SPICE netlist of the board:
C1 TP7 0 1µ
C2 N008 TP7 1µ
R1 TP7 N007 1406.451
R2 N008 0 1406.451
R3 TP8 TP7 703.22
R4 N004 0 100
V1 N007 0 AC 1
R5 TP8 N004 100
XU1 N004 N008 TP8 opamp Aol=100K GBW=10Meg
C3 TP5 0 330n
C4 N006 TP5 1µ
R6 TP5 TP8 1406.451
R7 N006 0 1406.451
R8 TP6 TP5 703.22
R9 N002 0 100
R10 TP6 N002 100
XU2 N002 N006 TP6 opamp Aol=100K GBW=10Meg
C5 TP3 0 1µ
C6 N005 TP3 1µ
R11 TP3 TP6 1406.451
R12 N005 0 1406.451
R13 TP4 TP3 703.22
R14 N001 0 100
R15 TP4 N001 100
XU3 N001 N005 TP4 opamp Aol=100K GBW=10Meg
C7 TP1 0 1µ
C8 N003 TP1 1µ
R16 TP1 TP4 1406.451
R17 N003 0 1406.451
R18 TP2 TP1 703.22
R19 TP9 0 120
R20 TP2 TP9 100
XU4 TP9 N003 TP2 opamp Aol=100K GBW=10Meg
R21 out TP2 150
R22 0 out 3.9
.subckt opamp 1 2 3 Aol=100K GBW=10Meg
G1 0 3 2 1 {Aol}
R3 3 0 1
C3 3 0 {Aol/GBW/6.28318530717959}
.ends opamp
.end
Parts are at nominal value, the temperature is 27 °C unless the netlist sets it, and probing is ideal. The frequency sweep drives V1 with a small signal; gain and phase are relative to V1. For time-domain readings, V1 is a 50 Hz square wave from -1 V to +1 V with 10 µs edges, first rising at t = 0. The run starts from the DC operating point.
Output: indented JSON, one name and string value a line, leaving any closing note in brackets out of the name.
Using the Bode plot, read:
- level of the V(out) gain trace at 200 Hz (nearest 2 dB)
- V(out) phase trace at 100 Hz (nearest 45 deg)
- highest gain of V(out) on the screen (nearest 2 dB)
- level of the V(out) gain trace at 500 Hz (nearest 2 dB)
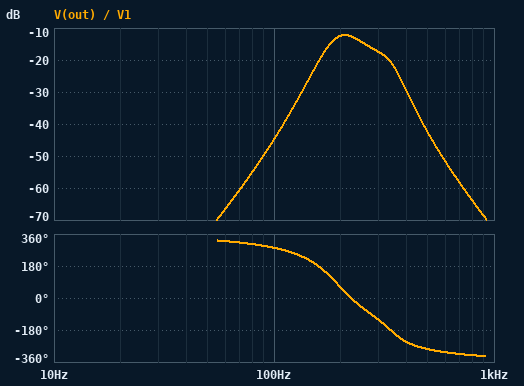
{
  "level of the V(out) gain trace at 200 Hz": "-12 dB",
  "V(out) phase trace at 100 Hz": "270 deg",
  "highest gain of V(out) on the screen": "-12 dB",
  "level of the V(out) gain trace at 500 Hz": "-42 dB"
}
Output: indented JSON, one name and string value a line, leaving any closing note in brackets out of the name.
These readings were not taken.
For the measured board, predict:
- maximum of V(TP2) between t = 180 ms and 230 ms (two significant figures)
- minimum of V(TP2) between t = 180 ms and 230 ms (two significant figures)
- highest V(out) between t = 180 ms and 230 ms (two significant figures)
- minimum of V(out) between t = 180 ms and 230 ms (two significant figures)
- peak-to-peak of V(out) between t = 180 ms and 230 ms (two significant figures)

{
  "maximum of V(TP2) between t = 180 ms and 230 ms": "3.1 V",
  "minimum of V(TP2) between t = 180 ms and 230 ms": "-3.1 V",
  "highest V(out) between t = 180 ms and 230 ms": "79 mV",
  "minimum of V(out) between t = 180 ms and 230 ms": "-79 mV",
  "peak-to-peak of V(out) between t = 180 ms and 230 ms": "160 mV"
}
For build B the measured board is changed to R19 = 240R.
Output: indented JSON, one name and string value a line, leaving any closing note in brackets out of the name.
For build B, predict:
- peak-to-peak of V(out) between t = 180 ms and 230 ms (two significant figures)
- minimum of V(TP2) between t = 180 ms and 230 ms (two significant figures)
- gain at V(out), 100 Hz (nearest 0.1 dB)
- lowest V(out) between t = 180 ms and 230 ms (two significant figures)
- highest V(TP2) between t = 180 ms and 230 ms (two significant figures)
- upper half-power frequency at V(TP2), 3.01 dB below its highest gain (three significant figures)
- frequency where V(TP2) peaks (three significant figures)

{
  "peak-to-peak of V(out) between t = 180 ms and 230 ms": "91 mV",
  "minimum of V(TP2) between t = 180 ms and 230 ms": "-1.8 V",
  "gain at V(out), 100 Hz": "-48.4 dB",
  "lowest V(out) between t = 180 ms and 230 ms": "-46 mV",
  "highest V(TP2) between t = 180 ms and 230 ms": "1.8 V",
  "upper half-power frequency at V(TP2), 3.01 dB below its highest gain": "286 Hz",
  "frequency where V(TP2) peaks": "213 Hz"
}
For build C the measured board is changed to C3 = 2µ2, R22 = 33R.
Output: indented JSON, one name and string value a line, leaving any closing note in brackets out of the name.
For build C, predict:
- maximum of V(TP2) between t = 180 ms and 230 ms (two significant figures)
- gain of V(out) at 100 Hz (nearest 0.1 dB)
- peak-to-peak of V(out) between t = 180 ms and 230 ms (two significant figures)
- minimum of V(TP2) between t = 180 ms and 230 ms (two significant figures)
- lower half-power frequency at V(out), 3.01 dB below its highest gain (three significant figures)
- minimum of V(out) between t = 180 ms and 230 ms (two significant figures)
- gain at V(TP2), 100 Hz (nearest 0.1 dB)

{
  "maximum of V(TP2) between t = 180 ms and 230 ms": "1.2 V",
  "gain of V(out) at 100 Hz": "-26.3 dB",
  "peak-to-peak of V(out) between t = 180 ms and 230 ms": "420 mV",
  "minimum of V(TP2) between t = 180 ms and 230 ms": "-1.2 V",
  "lower half-power frequency at V(out), 3.01 dB below its highest gain": "159 Hz",
  "minimum of V(out) between t = 180 ms and 230 ms": "-210 mV",
  "gain at V(TP2), 100 Hz": "-11.4 dB"
}
